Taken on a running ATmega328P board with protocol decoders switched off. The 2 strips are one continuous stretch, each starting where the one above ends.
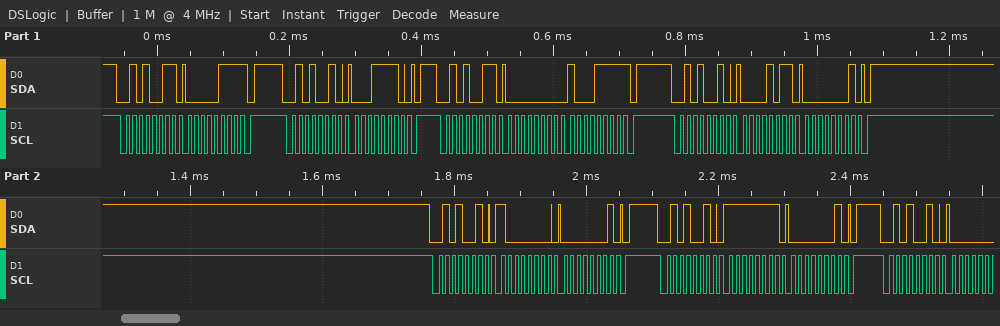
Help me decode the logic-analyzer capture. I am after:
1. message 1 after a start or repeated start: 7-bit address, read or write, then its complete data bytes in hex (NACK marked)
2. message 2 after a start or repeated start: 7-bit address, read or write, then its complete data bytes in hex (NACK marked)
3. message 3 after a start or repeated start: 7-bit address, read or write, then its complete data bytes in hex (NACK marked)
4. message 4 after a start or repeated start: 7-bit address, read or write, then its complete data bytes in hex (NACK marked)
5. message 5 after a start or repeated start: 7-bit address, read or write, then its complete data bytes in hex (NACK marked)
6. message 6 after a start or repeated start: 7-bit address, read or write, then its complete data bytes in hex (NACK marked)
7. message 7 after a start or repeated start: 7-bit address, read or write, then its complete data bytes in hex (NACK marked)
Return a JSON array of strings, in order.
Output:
["0x29 read: 07 NACK", "0x29 write: 1E", "0x29 read: 00 8F NACK", "0x29 write: 0B 01", "0x29 write: 80 01", "0x29 write: FF 01", "0x29 write"]
